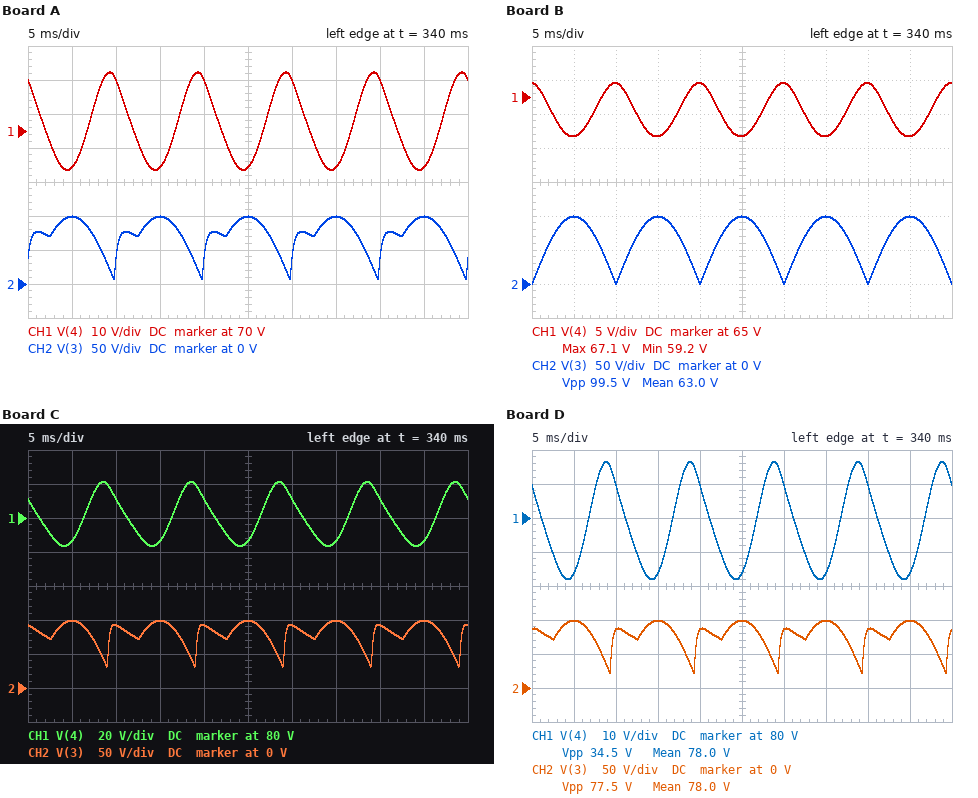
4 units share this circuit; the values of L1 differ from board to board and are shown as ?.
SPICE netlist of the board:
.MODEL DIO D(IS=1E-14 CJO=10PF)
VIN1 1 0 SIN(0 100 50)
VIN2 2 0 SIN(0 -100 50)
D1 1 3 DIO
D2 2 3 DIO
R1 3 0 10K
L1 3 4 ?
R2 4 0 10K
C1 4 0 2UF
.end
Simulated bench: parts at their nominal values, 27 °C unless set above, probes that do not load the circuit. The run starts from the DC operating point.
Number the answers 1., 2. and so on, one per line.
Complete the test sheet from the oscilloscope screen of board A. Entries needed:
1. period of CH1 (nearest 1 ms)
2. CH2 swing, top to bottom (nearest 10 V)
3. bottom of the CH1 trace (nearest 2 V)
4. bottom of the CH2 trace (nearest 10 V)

1. 10 ms
2. 90 V
3. 58 V
4. 10 V
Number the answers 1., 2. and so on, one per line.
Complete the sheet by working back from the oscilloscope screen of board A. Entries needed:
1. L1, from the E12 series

1. 3.9 H
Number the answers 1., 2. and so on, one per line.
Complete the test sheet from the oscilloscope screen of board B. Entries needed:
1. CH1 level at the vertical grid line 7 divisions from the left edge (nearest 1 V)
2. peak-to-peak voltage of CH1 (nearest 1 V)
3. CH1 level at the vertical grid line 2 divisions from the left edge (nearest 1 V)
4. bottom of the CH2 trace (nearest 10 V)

1. 59 V
2. 8 V
3. 67 V
4. 0 V
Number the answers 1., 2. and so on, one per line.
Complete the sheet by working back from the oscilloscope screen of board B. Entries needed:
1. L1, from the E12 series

1. 15 H
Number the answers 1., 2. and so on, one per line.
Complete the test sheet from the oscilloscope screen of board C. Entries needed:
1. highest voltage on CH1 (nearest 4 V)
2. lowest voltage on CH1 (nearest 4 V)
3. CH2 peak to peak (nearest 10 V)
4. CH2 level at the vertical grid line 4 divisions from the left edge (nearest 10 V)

1. 100 V
2. 64 V
3. 70 V
4. 90 V
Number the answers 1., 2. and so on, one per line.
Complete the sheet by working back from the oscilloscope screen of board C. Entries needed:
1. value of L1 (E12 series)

1. 2.2 H
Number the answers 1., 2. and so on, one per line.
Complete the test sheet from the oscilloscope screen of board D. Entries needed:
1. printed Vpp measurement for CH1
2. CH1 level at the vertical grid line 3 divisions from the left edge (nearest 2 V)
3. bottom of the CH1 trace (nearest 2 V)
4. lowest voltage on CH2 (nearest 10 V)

1. 34.5 V
2. 64 V
3. 62 V
4. 20 V
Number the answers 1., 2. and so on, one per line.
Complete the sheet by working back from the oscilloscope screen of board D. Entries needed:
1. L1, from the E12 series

1. 2.7 H
